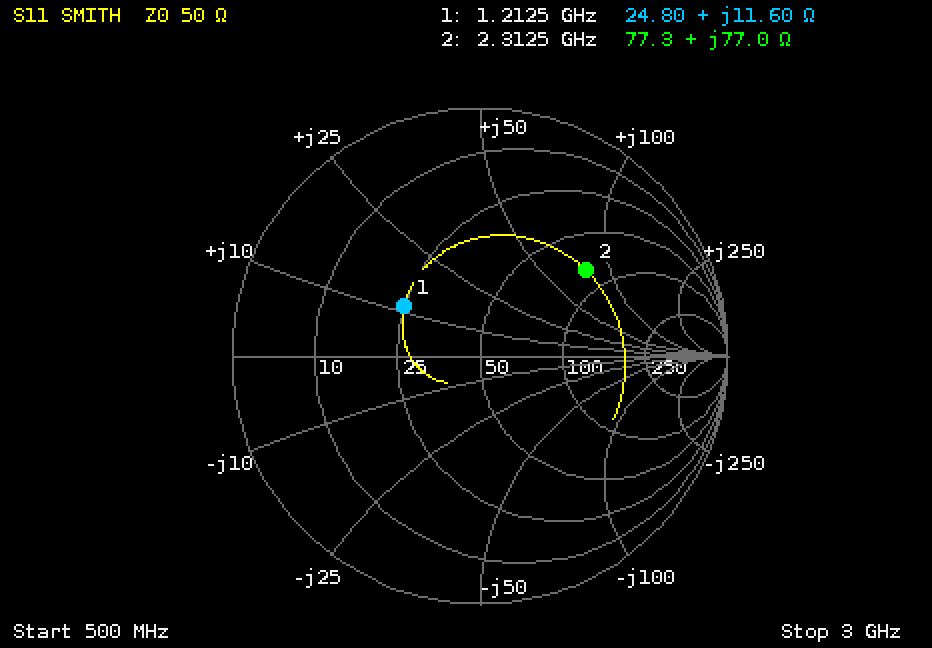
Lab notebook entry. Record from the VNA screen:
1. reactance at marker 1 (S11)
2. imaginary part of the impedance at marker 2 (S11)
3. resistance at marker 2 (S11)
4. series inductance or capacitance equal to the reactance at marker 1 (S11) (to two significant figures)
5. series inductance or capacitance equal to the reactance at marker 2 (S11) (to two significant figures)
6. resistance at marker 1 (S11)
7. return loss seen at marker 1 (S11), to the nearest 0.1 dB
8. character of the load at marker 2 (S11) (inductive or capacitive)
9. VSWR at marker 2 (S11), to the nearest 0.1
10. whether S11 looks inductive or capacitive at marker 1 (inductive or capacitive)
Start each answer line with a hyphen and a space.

- +11.60 Ω
- +77.0 Ω
- 77.3 Ω
- 1.5 nH
- 5.3 nH
- 24.80 Ω
- 8.7 dB
- inductive
- 3.4
- inductive
